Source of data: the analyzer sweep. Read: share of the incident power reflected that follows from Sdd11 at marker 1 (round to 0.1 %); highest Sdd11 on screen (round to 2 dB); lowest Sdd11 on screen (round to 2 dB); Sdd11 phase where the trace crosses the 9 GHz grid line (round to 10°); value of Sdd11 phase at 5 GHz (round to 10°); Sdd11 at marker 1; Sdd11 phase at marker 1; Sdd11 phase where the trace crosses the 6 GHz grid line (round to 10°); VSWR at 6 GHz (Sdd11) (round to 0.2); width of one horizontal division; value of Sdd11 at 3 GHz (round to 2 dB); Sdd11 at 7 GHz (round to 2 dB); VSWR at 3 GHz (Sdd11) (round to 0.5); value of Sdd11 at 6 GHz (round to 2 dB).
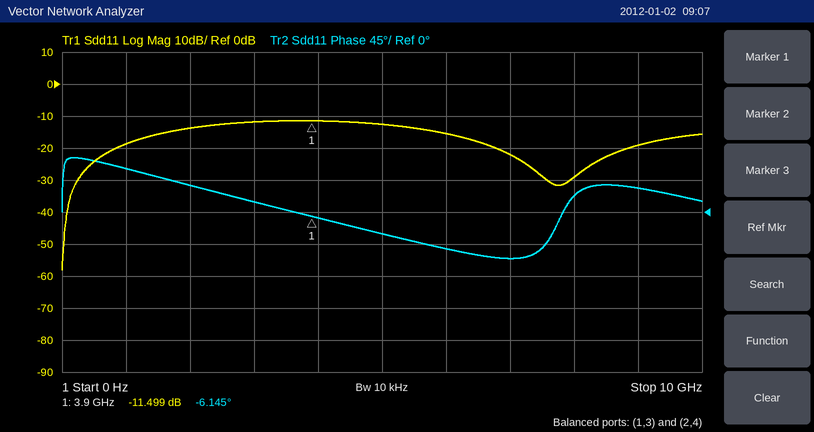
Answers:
7.1 %
-12 dB
-58 dB
30°
-30°
-11.499 dB
-6.145°
-50°
1.4
1 GHz
-12 dB
-22 dB
1.5
-16 dB
